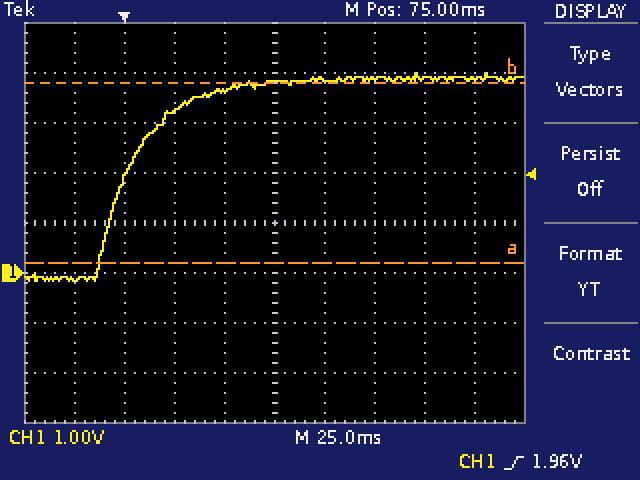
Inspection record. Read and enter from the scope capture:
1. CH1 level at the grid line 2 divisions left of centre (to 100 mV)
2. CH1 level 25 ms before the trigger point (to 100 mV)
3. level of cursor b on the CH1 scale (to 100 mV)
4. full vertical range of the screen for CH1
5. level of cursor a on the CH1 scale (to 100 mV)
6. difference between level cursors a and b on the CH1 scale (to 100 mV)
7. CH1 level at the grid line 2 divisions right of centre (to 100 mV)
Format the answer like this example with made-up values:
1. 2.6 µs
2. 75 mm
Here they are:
1. 3.2 V
2. -100 mV
3. 3.8 V
4. 8 V
5. 200 mV
6. 3.6 V
7. 3.9 V
